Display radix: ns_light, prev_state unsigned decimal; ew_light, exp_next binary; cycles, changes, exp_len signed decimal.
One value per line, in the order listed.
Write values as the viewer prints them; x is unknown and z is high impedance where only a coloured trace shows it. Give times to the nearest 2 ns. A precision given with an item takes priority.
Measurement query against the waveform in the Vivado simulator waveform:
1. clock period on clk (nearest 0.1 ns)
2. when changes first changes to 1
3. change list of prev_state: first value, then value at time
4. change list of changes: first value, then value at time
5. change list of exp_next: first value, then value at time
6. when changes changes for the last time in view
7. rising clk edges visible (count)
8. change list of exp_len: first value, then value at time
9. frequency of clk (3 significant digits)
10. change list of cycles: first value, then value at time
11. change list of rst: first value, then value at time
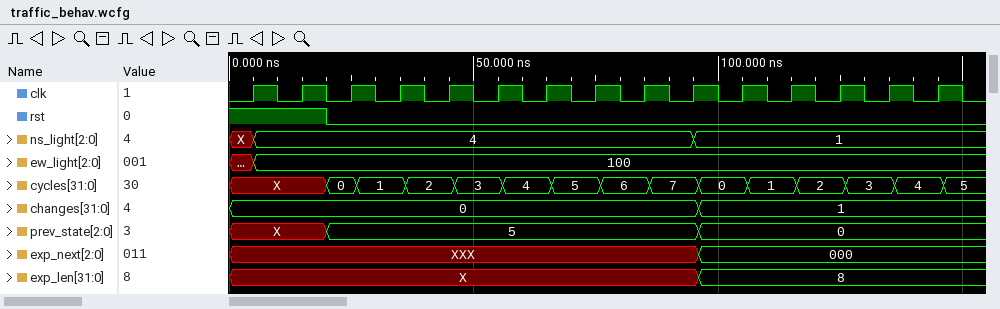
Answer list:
10 ns
96 ns
X, 5 at 20 ns, 0 at 96 ns
0, 1 at 96 ns
XXX, 000 at 96 ns
96 ns
15
X, 8 at 96 ns
100 MHz
X, 0 at 20 ns, 1 at 26 ns, 2 at 36 ns, 3 at 46 ns, 4 at 56 ns, 5 at 66 ns, 6 at 76 ns, 7 at 86 ns, 0 at 96 ns, 1 at 106 ns, 2 at 116 ns, 3 at 126 ns, 4 at 136 ns, 5 at 146 ns
1, 0 at 20 ns
